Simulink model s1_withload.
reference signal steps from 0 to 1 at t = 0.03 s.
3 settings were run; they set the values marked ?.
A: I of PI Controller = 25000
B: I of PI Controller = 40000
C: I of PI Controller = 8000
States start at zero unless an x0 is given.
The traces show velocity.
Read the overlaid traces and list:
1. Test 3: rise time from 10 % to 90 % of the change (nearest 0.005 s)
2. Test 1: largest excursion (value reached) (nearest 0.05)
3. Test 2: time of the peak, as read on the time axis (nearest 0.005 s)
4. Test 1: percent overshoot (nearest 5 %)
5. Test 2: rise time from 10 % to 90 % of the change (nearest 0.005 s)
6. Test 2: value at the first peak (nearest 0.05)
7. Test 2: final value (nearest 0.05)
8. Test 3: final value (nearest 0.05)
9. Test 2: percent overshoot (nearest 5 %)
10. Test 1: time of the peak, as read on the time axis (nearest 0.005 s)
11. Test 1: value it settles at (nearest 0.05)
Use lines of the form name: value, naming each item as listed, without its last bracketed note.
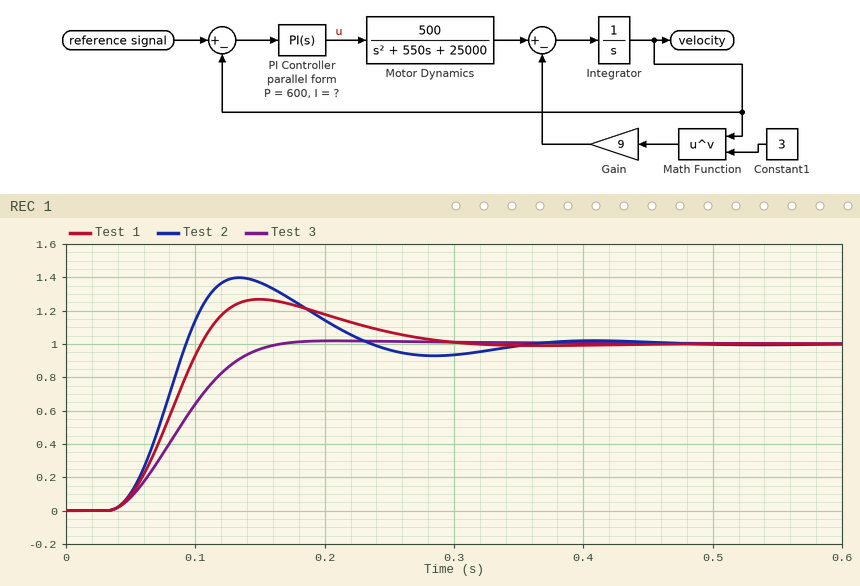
Test 3: rise time from 10 % to 90 % of the change: 0.080 s
Test 1: largest excursion (value reached): 1.25
Test 2: time of the peak, as read on the time axis: 0.135 s
Test 1: percent overshoot: 25 %
Test 2: rise time from 10 % to 90 % of the change: 0.040 s
Test 2: value at the first peak: 1.40
Test 2: final value: 1.00
Test 3: final value: 1.00
Test 2: percent overshoot: 40 %
Test 1: time of the peak, as read on the time axis: 0.150 s
Test 1: value it settles at: 1.00
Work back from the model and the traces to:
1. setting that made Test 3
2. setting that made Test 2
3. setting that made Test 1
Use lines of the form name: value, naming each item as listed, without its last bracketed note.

setting that made Test 3: C
setting that made Test 2: B
setting that made Test 1: A
